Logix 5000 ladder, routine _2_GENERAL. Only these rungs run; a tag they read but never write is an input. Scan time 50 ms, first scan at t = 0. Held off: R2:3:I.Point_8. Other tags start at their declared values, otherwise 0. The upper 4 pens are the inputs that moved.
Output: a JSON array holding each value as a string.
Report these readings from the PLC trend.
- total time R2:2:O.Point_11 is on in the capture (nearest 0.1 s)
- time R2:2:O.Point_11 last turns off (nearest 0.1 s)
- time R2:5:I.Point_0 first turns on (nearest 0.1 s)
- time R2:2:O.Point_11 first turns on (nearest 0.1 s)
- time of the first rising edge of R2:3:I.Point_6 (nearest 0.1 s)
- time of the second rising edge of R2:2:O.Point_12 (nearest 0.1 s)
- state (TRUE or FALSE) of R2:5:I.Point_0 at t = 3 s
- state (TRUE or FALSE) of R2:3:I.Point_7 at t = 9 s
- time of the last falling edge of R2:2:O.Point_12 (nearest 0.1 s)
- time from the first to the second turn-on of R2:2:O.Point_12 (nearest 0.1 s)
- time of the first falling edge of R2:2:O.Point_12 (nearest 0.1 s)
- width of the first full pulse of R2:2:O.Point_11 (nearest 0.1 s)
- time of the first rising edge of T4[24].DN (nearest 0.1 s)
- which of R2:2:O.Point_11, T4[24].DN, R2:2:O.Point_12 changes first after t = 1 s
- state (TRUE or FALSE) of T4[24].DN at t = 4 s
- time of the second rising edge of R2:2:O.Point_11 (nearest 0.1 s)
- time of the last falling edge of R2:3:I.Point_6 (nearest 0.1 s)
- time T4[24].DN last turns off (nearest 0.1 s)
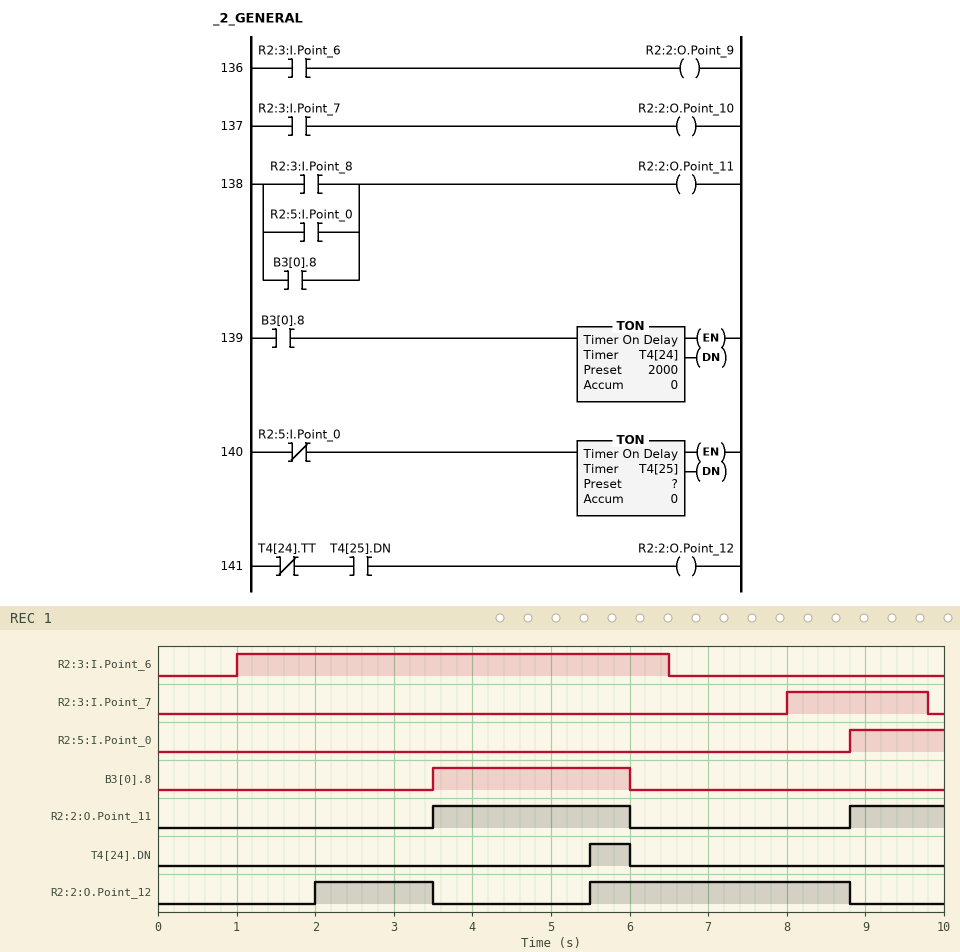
["3.7 s", "6.0 s", "8.8 s", "3.5 s", "1.0 s", "5.5 s", "FALSE", "TRUE", "8.8 s", "3.5 s", "3.5 s", "2.5 s", "5.5 s", "R2:2:O.Point_12", "FALSE", "8.8 s", "6.5 s", "6.0 s"]
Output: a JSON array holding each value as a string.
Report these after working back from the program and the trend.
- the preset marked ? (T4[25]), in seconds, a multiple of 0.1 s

["2.0 s"]
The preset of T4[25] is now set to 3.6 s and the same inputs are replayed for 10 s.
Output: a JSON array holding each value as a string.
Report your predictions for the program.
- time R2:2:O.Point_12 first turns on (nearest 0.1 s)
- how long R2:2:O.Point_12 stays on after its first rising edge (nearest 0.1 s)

["5.5 s", "3.3 s"]
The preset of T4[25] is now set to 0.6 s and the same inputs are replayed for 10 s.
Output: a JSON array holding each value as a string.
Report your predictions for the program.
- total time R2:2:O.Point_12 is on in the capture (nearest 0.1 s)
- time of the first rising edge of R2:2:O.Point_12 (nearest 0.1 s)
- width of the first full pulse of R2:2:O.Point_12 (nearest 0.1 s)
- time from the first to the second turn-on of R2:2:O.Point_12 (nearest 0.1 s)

["6.2 s", "0.6 s", "2.9 s", "4.9 s"]
